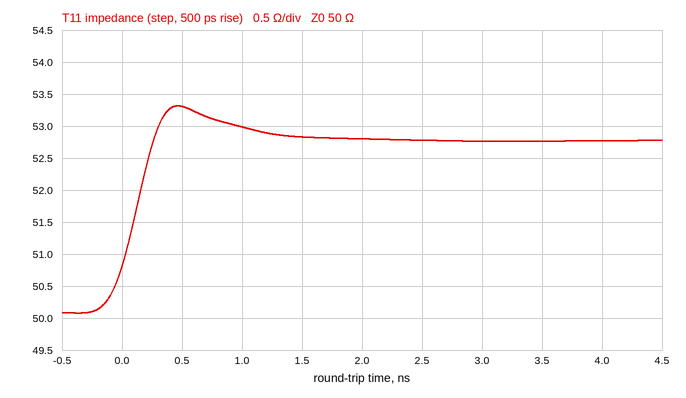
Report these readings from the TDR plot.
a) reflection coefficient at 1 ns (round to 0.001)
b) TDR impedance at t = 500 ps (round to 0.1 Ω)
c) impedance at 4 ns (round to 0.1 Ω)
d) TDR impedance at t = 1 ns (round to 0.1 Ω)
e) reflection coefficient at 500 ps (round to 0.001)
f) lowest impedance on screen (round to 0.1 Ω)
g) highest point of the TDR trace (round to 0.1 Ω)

+0.029
53.3 Ω
52.8 Ω
53.0 Ω
+0.032
50.1 Ω
53.3 Ω
